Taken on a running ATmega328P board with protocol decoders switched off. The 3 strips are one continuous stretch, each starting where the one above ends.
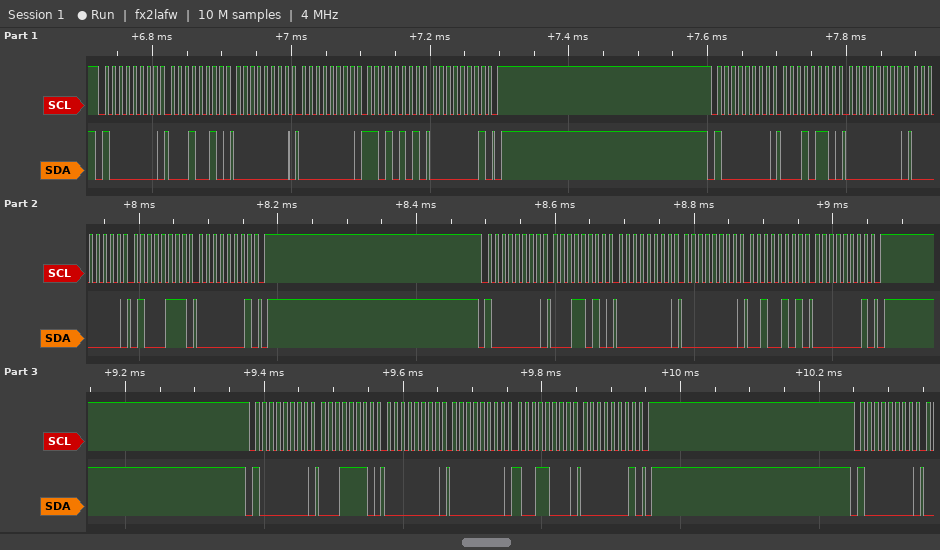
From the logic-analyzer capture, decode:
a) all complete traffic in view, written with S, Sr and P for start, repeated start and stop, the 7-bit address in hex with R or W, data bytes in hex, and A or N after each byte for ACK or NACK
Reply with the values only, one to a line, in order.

S 40W A 12 A 00 A 00 A D5 A 01 A P S 40W A 16 A 00 A 00 A 47 A 01 A P S 40W A 1A A 00 A 00 A 25 A 01 A P S 40W A 1E A 00 A 00 A 98 A 01 A P S 40W A
